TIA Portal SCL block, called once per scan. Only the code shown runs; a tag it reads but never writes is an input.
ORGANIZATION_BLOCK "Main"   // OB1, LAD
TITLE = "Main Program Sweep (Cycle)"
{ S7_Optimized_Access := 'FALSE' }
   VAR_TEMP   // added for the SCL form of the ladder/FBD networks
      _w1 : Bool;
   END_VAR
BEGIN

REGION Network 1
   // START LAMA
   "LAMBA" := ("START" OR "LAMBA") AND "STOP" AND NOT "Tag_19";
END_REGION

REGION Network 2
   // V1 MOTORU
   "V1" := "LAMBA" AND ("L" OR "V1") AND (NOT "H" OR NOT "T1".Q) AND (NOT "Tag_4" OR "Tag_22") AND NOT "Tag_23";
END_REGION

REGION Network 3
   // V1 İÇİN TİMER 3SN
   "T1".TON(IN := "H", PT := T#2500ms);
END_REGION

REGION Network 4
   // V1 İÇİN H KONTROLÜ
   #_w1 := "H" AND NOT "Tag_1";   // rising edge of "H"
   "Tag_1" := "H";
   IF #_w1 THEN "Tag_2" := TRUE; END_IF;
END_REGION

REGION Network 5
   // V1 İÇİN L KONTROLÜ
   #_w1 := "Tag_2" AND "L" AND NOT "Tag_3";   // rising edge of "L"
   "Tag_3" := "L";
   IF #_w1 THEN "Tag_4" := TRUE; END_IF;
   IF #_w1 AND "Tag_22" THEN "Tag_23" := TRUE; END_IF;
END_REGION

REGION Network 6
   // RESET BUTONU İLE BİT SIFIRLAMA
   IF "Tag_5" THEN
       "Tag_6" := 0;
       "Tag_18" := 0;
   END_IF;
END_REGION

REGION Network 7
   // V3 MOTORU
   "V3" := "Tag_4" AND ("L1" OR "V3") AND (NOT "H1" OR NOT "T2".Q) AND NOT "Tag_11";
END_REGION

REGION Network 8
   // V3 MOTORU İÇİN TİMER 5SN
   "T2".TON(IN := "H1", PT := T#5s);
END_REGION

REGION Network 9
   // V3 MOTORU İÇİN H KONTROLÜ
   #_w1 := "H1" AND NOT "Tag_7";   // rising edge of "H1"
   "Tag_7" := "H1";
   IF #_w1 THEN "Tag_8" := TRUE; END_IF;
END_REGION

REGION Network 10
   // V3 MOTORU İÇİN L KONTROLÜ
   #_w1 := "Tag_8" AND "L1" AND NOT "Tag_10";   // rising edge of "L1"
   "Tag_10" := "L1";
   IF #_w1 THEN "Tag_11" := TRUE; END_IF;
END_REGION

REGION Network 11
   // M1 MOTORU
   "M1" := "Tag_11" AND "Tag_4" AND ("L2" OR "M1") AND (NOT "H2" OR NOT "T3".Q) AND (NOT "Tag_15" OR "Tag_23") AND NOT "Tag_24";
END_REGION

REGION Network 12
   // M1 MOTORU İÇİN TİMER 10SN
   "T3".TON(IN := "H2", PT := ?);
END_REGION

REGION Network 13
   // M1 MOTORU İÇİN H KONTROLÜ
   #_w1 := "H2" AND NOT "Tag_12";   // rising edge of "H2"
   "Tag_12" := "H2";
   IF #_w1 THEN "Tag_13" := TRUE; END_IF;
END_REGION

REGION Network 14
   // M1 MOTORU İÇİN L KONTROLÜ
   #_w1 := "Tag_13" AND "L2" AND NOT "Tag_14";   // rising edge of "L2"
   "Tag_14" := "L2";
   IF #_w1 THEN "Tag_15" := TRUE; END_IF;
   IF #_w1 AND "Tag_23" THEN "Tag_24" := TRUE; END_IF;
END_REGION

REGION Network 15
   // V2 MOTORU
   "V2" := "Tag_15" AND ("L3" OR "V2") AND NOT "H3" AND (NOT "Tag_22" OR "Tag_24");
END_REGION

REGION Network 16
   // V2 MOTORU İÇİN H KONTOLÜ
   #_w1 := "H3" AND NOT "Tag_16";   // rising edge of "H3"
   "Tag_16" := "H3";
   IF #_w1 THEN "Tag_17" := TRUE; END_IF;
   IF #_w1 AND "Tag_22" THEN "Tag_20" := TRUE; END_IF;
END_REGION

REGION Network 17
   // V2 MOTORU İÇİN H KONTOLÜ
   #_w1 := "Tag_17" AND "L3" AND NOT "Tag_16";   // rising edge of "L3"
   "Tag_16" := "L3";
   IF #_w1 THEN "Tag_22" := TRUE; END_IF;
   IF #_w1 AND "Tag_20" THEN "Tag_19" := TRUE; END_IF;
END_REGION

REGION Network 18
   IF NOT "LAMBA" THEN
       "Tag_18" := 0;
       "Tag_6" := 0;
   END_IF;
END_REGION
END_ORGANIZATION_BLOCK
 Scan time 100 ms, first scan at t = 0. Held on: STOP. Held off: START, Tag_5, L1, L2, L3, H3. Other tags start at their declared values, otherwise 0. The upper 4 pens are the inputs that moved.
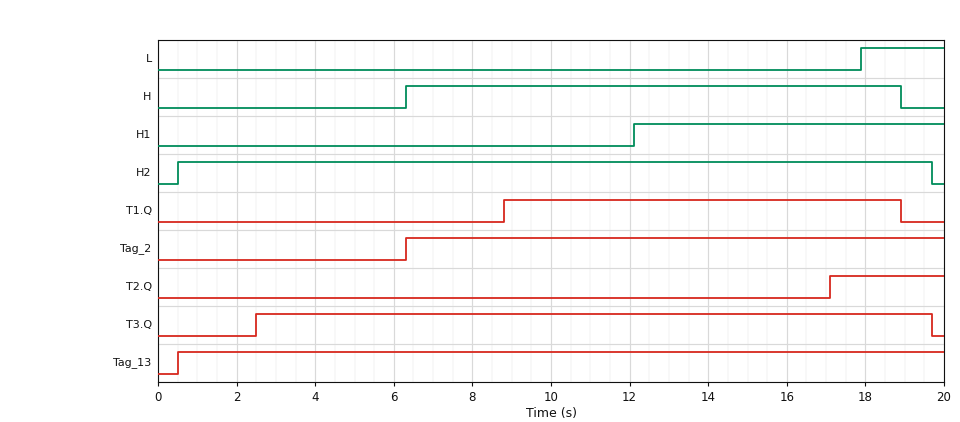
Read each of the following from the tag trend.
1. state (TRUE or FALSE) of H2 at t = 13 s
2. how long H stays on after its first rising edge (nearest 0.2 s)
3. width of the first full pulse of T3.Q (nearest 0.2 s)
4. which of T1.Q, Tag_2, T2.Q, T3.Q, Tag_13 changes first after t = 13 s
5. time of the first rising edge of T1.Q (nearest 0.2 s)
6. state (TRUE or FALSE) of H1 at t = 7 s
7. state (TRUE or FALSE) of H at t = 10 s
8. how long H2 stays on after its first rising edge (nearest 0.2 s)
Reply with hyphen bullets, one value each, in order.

- TRUE
- 12.6 s
- 17.2 s
- T2.Q
- 8.8 s
- FALSE
- TRUE
- 19.2 s
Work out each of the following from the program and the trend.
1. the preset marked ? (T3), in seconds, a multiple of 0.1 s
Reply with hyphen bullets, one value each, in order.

- 2.0 s
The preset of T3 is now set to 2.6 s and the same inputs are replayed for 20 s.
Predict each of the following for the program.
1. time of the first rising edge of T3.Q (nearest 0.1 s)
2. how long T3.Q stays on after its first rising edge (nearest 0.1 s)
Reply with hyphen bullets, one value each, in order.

- 3.1 s
- 16.6 s
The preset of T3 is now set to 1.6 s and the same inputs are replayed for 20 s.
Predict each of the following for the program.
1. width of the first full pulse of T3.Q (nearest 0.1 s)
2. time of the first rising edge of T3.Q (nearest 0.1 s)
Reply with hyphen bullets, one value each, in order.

- 17.6 s
- 2.1 s
